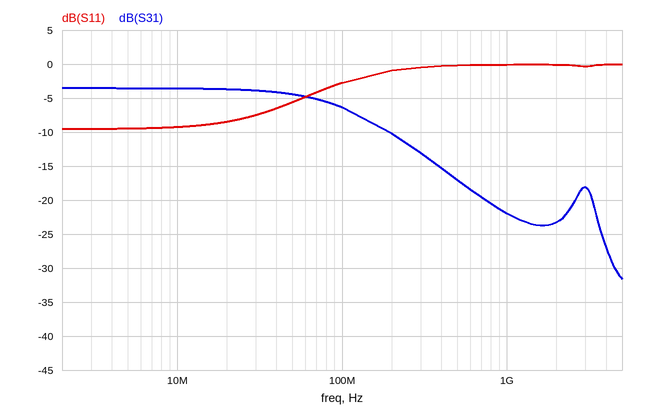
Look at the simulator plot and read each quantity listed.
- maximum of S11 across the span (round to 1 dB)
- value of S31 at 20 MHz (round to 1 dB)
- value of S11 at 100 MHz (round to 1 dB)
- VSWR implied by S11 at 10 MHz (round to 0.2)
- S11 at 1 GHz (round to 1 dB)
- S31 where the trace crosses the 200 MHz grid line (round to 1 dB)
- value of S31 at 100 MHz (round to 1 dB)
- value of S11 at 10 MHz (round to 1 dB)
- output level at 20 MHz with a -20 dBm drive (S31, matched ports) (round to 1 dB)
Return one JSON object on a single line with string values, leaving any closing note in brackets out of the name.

{"maximum of S11 across the span": "0 dB", "value of S31 at 20 MHz": "-4 dB", "value of S11 at 100 MHz": "-3 dB", "VSWR implied by S11 at 10 MHz": "2.0", "S11 at 1 GHz": "0 dB", "S31 where the trace crosses the 200 MHz grid line": "-10 dB", "value of S31 at 100 MHz": "-6 dB", "value of S11 at 10 MHz": "-9 dB", "output level at 20 MHz with a -20 dBm drive (S31, matched ports)": "-24 dBm"}
